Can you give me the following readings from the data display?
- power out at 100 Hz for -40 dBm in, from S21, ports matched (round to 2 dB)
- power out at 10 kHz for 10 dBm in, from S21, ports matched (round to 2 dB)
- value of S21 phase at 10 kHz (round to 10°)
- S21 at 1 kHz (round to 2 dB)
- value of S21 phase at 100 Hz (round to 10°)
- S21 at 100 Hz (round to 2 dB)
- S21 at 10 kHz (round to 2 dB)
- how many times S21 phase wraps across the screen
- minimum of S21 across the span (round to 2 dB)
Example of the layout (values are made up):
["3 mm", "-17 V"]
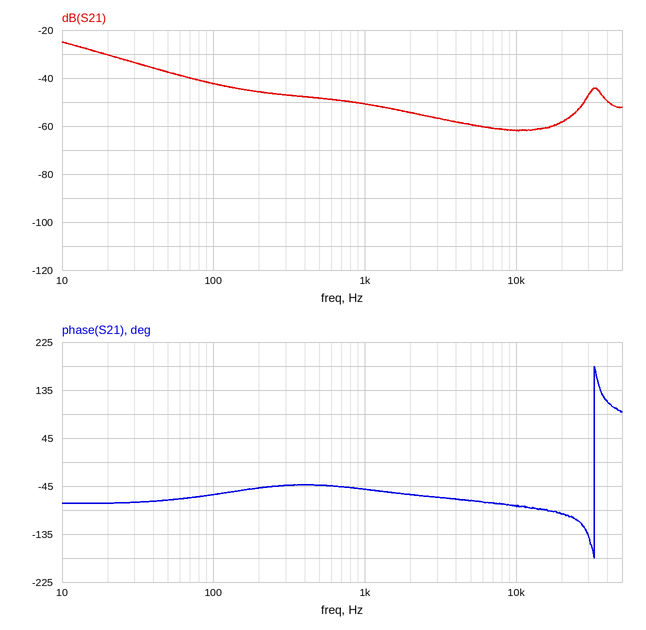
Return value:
["-82 dBm", "-52 dBm", "-80°", "-50 dB", "-60°", "-42 dB", "-62 dB", "1", "-62 dB"]
